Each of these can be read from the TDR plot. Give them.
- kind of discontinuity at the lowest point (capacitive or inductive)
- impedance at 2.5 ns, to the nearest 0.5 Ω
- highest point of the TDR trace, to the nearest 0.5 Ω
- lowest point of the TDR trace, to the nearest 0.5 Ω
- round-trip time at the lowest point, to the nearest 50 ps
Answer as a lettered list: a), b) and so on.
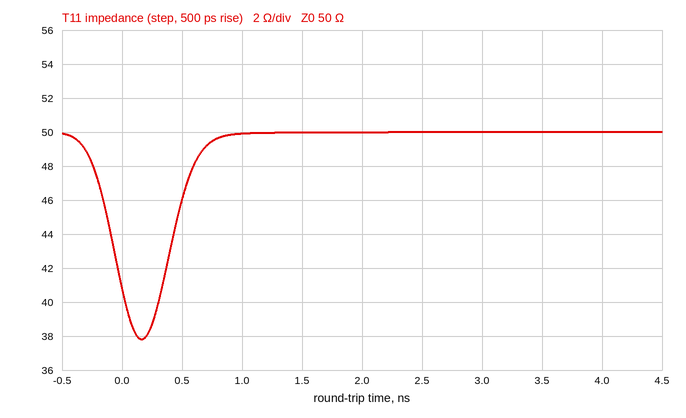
a) capacitive
b) 50.0 Ω
c) 50.0 Ω
d) 38.0 Ω
e) 150 ps
